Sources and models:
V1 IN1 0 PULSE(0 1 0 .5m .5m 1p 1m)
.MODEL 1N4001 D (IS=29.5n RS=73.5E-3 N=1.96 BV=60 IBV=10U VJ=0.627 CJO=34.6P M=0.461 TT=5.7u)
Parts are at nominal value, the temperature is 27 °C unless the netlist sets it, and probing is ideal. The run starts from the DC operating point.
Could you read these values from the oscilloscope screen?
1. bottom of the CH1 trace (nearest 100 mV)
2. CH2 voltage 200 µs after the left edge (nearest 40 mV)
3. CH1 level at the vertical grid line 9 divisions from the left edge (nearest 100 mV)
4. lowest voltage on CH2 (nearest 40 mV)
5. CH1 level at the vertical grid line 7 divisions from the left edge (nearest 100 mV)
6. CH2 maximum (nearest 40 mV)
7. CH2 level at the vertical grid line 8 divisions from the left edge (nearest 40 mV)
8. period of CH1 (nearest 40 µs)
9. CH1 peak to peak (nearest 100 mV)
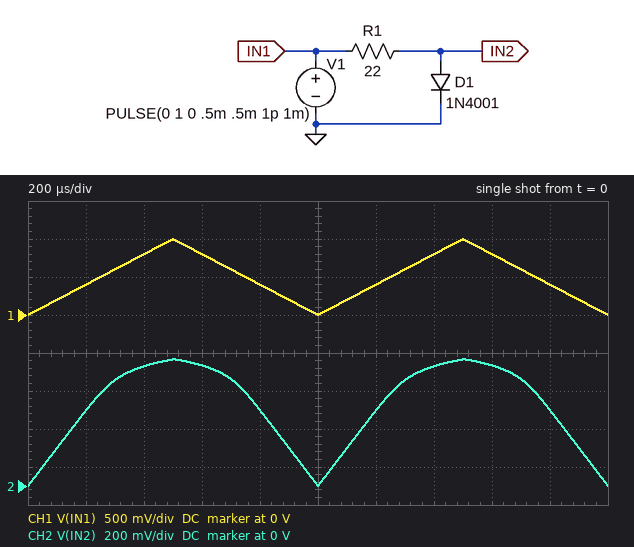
0 V
400 mV
400 mV
0 V
800 mV
680 mV
640 mV
1.00 ms
1.0 V
